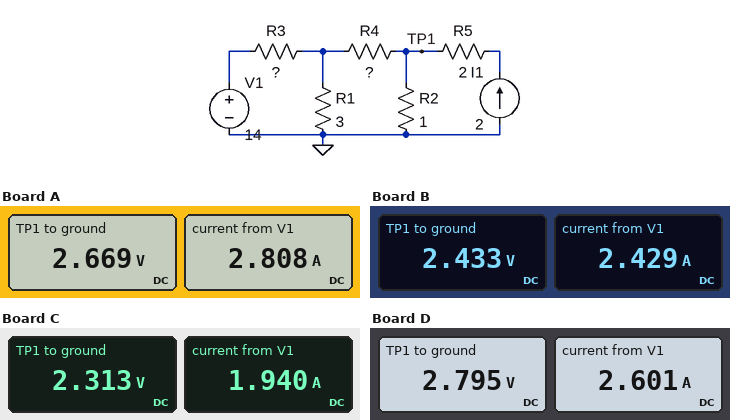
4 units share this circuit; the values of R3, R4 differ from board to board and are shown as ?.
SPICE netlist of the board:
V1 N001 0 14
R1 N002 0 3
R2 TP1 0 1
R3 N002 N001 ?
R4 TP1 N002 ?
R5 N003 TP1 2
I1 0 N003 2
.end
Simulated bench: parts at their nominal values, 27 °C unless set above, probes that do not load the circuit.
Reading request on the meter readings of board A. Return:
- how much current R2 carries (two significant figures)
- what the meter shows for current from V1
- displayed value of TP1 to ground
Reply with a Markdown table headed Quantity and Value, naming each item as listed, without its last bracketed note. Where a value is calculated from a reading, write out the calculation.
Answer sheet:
| Quantity | Value |
|---|---|
| how much current R2 carries | (2.669 V) / 1 Ω = 2.7 A |
| what the meter shows for current from V1 | 2.808 A |
| displayed value of TP1 to ground | 2.669 V |
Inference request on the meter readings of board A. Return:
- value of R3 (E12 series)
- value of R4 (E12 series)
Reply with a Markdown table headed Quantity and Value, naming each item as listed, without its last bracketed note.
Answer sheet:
| Quantity | Value |
|---|---|
| value of R3 | 2.7 Ω |
| value of R4 | 5.6 Ω |
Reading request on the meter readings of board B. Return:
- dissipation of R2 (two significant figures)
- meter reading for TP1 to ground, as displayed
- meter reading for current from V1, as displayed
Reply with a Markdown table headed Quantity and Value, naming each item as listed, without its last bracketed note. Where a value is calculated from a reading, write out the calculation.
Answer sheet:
| Quantity | Value |
|---|---|
| dissipation of R2 | (2.433 V)^2 / 1 Ω = 5.9 W |
| meter reading for TP1 to ground, as displayed | 2.433 V |
| meter reading for current from V1, as displayed | 2.429 A |
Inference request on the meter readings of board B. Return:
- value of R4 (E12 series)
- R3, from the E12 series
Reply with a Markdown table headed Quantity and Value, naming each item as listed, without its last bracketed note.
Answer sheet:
| Quantity | Value |
|---|---|
| value of R4 | 8.2 Ω |
| R3, from the E12 series | 3.3 Ω |
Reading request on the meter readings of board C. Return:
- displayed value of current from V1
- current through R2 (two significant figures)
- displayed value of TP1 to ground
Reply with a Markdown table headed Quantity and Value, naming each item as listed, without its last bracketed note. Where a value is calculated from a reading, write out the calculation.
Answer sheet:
| Quantity | Value |
|---|---|
| displayed value of current from V1 | 1.940 A |
| current through R2 | (2.313 V) / 1 Ω = 2.3 A |
| displayed value of TP1 to ground | 2.313 V |
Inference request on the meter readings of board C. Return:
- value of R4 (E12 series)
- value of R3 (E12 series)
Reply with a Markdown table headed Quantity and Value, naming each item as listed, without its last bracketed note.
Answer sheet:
| Quantity | Value |
|---|---|
| value of R4 | 8.2 Ω |
| value of R3 | 4.7 Ω |
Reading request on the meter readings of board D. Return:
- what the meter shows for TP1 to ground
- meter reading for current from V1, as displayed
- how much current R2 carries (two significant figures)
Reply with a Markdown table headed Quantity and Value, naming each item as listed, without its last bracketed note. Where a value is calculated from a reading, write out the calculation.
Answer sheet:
| Quantity | Value |
|---|---|
| what the meter shows for TP1 to ground | 2.795 V |
| meter reading for current from V1, as displayed | 2.601 A |
| how much current R2 carries | (2.795 V) / 1 Ω = 2.8 A |
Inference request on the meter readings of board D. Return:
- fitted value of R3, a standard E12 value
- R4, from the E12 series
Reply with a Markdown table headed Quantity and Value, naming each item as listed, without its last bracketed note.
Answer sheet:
| Quantity | Value |
|---|---|
| fitted value of R3, a standard E12 value | 3.3 Ω |
| R4, from the E12 series | 3.3 Ω |
